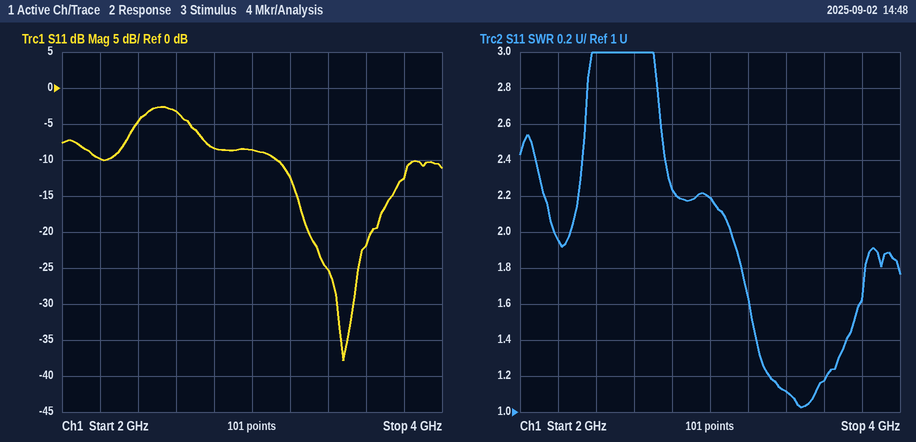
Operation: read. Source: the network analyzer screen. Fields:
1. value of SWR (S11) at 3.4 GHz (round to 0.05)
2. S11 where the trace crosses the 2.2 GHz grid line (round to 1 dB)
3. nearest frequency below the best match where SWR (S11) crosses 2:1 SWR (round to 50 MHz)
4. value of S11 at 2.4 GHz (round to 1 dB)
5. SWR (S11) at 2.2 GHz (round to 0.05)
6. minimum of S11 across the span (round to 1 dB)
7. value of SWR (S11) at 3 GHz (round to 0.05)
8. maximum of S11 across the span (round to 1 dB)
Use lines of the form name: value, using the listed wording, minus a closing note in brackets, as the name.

value of SWR (S11) at 3.4 GHz: 1.10
S11 where the trace crosses the 2.2 GHz grid line: -10 dB
nearest frequency below the best match where SWR (S11) crosses 2:1 SWR: 3.10 GHz
value of S11 at 2.4 GHz: -5 dB
SWR (S11) at 2.2 GHz: 1.95
minimum of S11 across the span: -38 dB
value of SWR (S11) at 3 GHz: 2.20
maximum of S11 across the span: -3 dB
